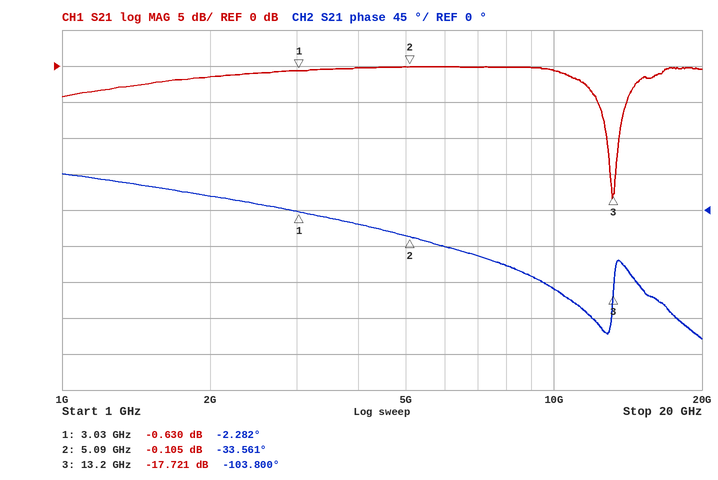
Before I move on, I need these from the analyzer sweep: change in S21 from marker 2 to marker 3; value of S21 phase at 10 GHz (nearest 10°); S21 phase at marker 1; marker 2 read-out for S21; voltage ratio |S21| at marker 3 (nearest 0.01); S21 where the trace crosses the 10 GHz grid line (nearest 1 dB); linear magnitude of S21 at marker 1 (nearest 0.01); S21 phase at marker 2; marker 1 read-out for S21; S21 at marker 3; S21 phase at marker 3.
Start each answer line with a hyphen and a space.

- -17.616 dB
- -100°
- -2.282°
- -0.105 dB
- 0.13
- -1 dB
- 0.93
- -33.561°
- -0.630 dB
- -17.721 dB
- -103.800°
